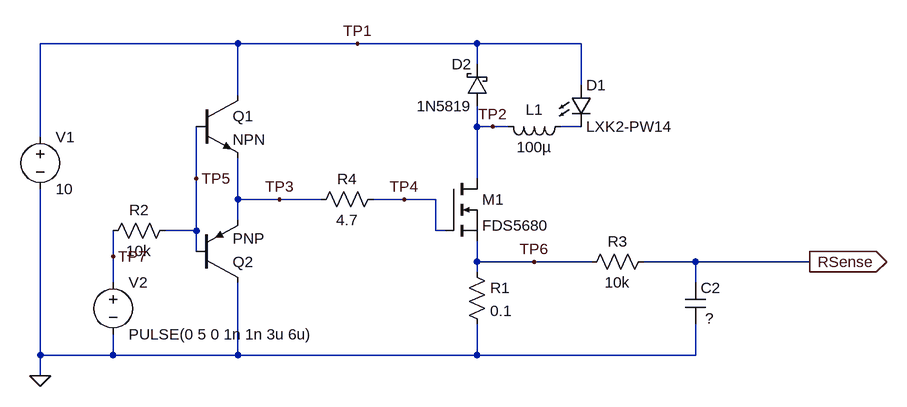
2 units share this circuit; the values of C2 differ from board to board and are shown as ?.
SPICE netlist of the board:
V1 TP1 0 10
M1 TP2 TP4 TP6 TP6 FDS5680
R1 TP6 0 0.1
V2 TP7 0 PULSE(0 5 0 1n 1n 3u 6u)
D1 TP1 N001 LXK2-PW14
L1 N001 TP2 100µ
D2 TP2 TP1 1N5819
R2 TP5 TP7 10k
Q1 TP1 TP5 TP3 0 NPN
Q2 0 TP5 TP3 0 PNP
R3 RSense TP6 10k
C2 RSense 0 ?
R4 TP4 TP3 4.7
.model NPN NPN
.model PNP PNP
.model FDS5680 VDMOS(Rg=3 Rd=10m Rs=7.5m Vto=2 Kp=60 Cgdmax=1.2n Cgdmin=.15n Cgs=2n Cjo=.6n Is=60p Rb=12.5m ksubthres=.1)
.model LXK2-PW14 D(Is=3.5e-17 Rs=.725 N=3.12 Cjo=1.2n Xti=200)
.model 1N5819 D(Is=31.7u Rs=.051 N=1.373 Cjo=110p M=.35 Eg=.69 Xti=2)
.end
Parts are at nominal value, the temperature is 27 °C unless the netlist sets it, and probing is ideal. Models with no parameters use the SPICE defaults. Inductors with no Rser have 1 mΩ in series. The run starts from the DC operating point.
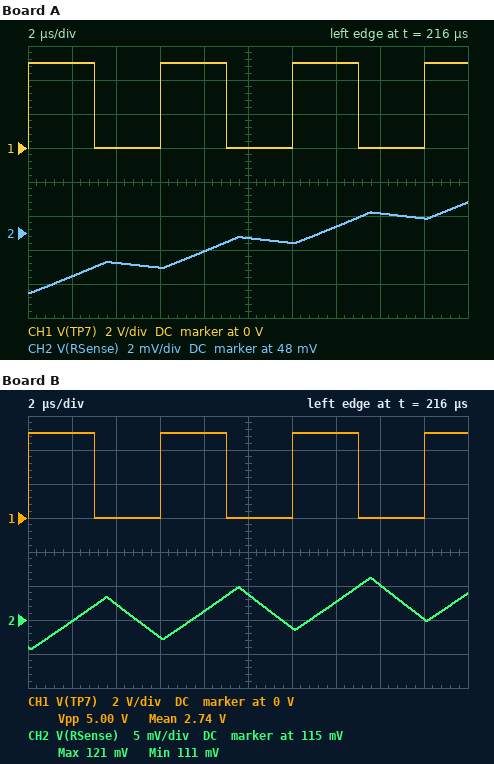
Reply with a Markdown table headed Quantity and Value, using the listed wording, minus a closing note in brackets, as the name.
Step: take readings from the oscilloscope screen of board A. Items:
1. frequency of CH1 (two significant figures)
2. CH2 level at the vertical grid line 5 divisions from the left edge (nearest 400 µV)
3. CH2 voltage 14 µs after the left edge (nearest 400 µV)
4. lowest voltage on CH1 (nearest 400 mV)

| Quantity | Value |
|---|---|
| frequency of CH1 | 170 kHz |
| CH2 level at the vertical grid line 5 divisions from the left edge | 47.6 mV |
| CH2 voltage 14 µs after the left edge | 48.4 mV |
| lowest voltage on CH1 | 0 V |
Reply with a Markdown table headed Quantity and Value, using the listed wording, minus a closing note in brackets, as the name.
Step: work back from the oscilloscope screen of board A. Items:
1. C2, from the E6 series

| Quantity | Value |
|---|---|
| C2, from the E6 series | 33 nF |
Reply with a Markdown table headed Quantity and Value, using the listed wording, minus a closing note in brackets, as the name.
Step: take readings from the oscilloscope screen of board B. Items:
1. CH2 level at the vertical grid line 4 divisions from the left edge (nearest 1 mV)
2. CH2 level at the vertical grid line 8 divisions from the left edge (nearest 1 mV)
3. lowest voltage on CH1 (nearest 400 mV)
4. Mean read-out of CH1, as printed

| Quantity | Value |
|---|---|
| CH2 level at the vertical grid line 4 divisions from the left edge | 116 mV |
| CH2 level at the vertical grid line 8 divisions from the left edge | 120 mV |
| lowest voltage on CH1 | 0 V |
| Mean read-out of CH1, as printed | 2.74 V |
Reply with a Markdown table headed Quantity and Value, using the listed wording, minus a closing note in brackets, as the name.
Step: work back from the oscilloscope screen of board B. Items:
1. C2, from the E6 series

| Quantity | Value |
|---|---|
| C2, from the E6 series | 4.7 nF |
